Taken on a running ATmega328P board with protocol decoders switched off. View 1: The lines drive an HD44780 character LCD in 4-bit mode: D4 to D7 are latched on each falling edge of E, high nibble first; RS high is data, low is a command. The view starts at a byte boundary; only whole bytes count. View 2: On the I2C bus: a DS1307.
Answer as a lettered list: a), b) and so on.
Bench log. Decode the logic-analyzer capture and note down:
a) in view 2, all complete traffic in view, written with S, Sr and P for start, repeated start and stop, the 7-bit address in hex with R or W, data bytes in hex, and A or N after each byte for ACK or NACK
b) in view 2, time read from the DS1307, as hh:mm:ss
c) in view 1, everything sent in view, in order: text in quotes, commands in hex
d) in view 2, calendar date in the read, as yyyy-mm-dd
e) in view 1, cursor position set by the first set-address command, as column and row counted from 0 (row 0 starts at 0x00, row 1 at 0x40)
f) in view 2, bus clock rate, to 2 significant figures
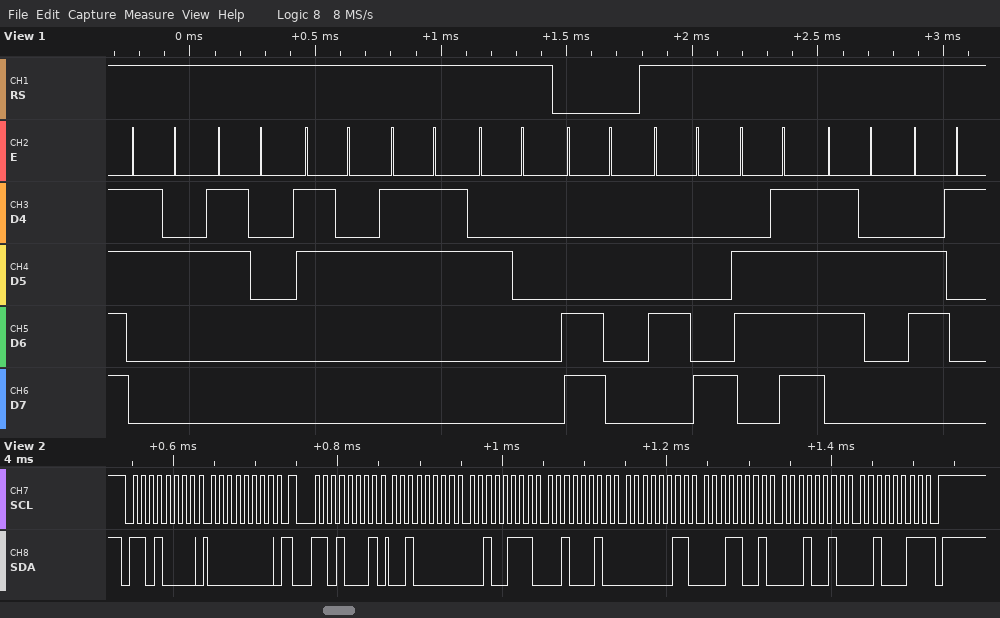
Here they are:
a) S 68W A 00 A Sr 68R A 20 A 27 A 22 A 03 A 19 A 12 A 23 N P
b) 22:27:20
c) "2023 " 0xC0 "Hora"
d) 2023-12-19
e) column 0, row 1
f) 100 kHz
